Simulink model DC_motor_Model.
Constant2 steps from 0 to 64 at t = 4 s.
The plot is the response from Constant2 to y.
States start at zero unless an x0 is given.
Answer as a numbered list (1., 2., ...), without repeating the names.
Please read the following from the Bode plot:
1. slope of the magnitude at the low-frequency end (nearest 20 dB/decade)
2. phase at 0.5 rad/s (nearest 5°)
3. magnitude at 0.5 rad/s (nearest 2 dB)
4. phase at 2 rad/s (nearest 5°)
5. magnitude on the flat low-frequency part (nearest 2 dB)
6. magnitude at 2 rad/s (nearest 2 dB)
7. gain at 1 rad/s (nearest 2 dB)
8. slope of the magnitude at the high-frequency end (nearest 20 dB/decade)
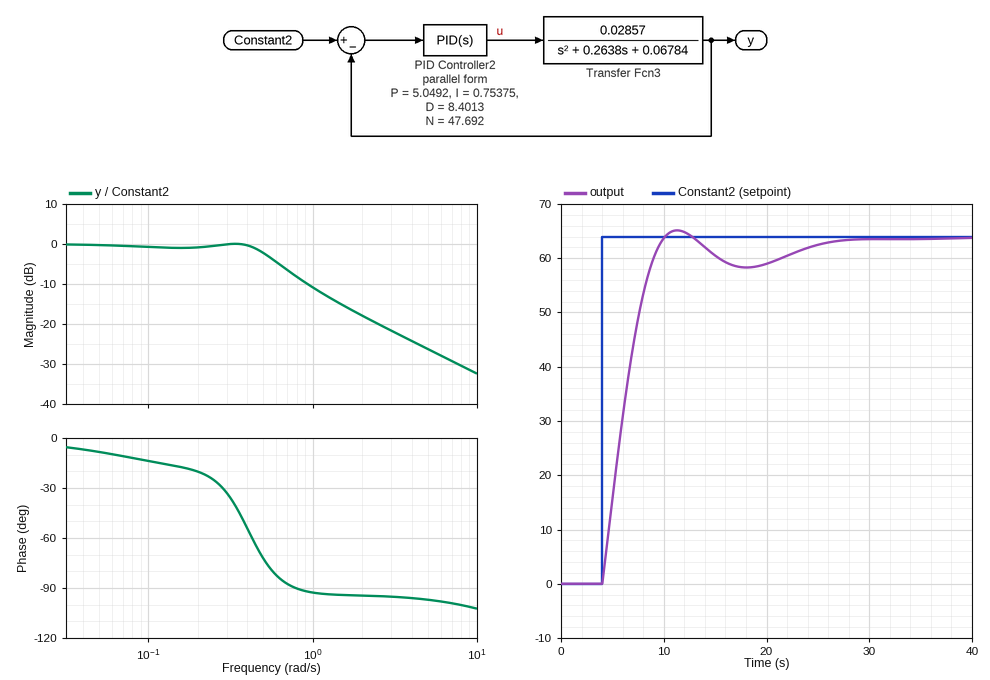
1. 0 dB/decade
2. -70°
3. -2 dB
4. -95°
5. 0 dB
6. -18 dB
7. -10 dB
8. -20 dB/decade
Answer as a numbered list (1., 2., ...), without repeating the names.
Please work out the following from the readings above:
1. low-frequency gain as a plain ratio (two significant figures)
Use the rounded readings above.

1. 1.0
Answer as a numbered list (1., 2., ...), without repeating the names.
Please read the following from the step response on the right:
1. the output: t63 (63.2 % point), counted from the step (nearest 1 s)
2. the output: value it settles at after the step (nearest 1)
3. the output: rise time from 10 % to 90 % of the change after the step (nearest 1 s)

1. 3 s
2. 64
3. 4 s
